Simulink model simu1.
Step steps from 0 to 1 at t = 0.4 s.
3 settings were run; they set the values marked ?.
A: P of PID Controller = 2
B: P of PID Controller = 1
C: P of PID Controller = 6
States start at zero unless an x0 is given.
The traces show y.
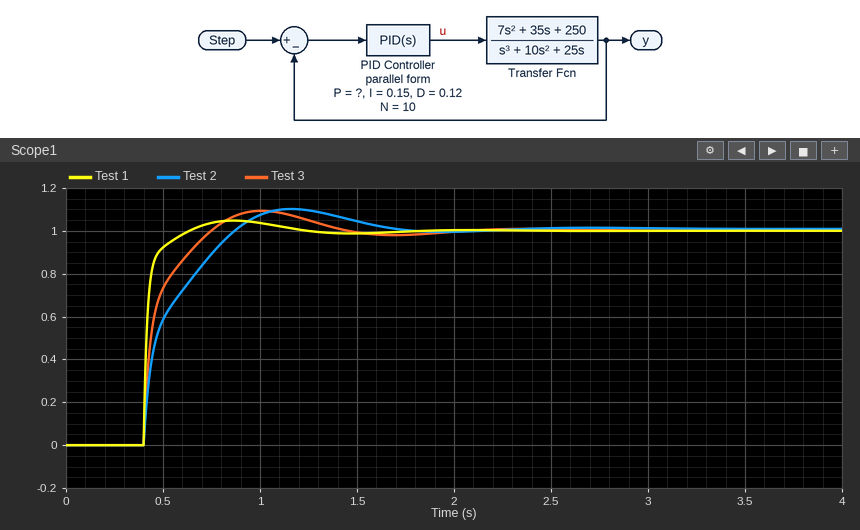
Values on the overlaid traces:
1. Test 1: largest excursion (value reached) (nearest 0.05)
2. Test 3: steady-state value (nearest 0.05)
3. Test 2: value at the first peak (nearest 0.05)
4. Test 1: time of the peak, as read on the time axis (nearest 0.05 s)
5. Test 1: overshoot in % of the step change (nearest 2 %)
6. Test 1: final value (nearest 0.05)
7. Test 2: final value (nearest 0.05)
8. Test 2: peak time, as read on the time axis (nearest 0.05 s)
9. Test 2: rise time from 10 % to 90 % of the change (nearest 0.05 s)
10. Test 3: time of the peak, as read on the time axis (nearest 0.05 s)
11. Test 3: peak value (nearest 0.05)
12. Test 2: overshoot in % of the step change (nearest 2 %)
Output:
1.05
1.00
1.10
0.85 s
4 %
1.00
1.00
1.15 s
0.35 s
1.00 s
1.10
10 %
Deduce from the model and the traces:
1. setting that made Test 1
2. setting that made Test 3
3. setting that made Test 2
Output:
C
A
B
